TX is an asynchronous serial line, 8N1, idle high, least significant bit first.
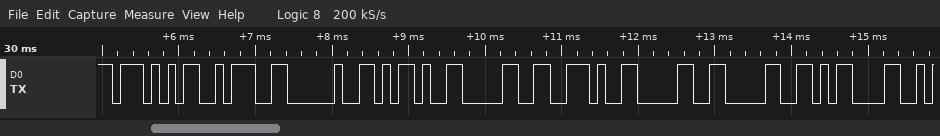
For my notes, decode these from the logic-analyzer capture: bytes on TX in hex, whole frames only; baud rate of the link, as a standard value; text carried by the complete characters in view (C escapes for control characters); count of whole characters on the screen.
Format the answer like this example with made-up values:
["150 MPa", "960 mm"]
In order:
["0x57 0x3A 0x20 0x2D 0x30 0x2E 0x30 0x30 0x0D", "9600 baud", "\"W: -0.00\\r\"", "9"]
